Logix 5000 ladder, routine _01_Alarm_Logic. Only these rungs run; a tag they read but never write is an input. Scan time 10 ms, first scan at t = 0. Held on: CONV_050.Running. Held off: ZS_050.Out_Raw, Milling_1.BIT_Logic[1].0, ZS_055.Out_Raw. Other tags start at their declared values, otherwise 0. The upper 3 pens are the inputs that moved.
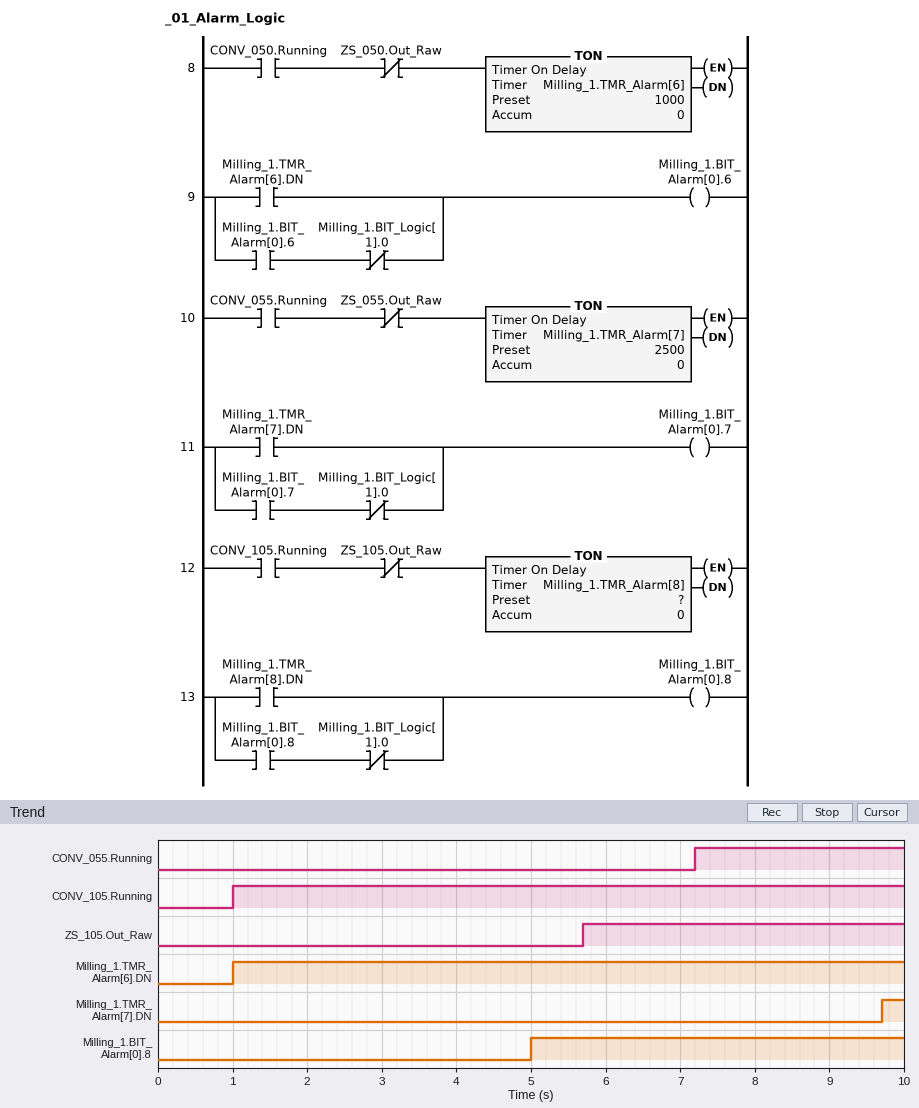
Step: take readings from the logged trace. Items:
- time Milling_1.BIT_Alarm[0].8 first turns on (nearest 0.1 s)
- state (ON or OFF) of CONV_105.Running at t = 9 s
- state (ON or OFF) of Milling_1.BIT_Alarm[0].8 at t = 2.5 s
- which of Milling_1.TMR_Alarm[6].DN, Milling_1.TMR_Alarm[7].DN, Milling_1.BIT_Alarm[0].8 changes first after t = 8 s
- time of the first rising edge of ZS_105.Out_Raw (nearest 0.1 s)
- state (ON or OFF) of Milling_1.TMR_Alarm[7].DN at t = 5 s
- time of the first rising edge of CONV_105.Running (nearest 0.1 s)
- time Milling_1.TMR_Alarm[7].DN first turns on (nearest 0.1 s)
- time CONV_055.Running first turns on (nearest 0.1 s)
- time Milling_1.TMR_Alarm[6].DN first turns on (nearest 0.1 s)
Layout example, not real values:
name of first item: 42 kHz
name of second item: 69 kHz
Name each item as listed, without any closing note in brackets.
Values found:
time Milling_1.BIT_Alarm[0].8 first turns on: 5.0 s
state (ON or OFF) of CONV_105.Running at t = 9 s: ON
state (ON or OFF) of Milling_1.BIT_Alarm[0].8 at t = 2.5 s: OFF
which of Milling_1.TMR_Alarm[6].DN, Milling_1.TMR_Alarm[7].DN, Milling_1.BIT_Alarm[0].8 changes first after t = 8 s: Milling_1.TMR_Alarm[7].DN
time of the first rising edge of ZS_105.Out_Raw: 5.7 s
state (ON or OFF) of Milling_1.TMR_Alarm[7].DN at t = 5 s: OFF
time of the first rising edge of CONV_105.Running: 1.0 s
time Milling_1.TMR_Alarm[7].DN first turns on: 9.7 s
time CONV_055.Running first turns on: 7.2 s
time Milling_1.TMR_Alarm[6].DN first turns on: 1.0 s
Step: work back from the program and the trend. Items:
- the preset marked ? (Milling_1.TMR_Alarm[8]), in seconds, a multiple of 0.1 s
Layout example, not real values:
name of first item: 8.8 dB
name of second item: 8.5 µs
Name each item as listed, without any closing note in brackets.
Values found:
the preset marked ? (Milling_1.TMR_Alarm[8]), in seconds, a multiple of 0.1 s: 4.0 s
